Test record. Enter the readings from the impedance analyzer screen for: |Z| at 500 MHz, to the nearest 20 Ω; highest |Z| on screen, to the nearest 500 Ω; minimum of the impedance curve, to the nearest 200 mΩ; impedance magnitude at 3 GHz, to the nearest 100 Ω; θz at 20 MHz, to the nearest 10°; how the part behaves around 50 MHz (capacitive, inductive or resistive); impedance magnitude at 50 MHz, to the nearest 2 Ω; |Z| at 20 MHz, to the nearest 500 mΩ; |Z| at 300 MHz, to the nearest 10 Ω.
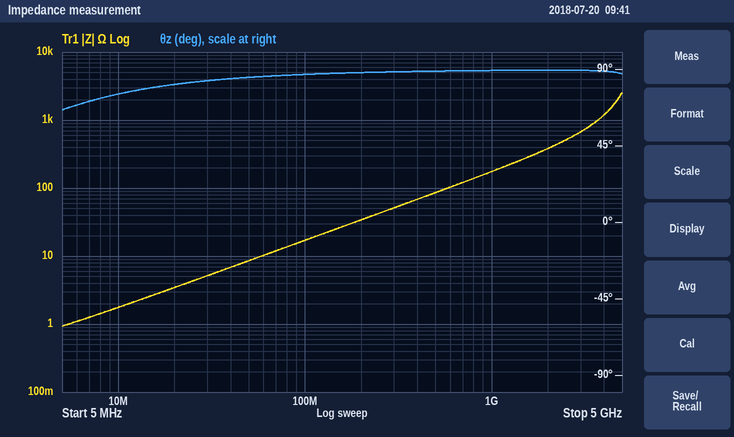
80 Ω
2.5 kΩ
1.0 Ω
700 Ω
80°
inductive
8 Ω
3.5 Ω
50 Ω
